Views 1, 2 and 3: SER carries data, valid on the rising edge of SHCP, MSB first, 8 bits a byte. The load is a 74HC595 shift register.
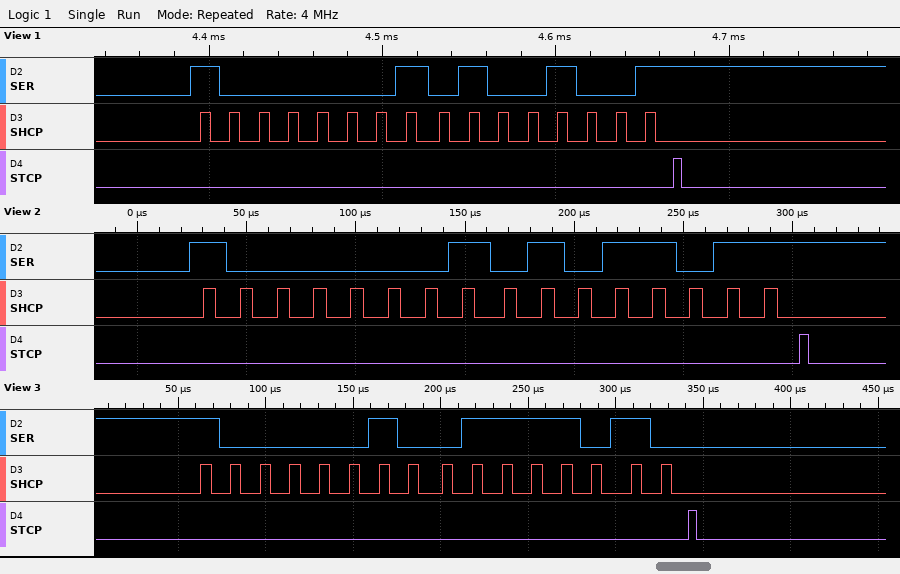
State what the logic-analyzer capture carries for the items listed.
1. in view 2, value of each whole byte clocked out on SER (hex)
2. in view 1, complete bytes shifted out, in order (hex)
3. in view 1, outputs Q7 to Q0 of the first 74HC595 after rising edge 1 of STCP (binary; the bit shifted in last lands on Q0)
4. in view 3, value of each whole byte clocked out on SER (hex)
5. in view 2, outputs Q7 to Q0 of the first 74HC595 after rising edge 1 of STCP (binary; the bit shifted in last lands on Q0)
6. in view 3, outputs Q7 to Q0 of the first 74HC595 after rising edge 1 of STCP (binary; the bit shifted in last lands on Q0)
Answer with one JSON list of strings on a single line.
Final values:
["81 5B", "81 49", "01001001", "0x82 0x7A", "01011011", "01111010"]
